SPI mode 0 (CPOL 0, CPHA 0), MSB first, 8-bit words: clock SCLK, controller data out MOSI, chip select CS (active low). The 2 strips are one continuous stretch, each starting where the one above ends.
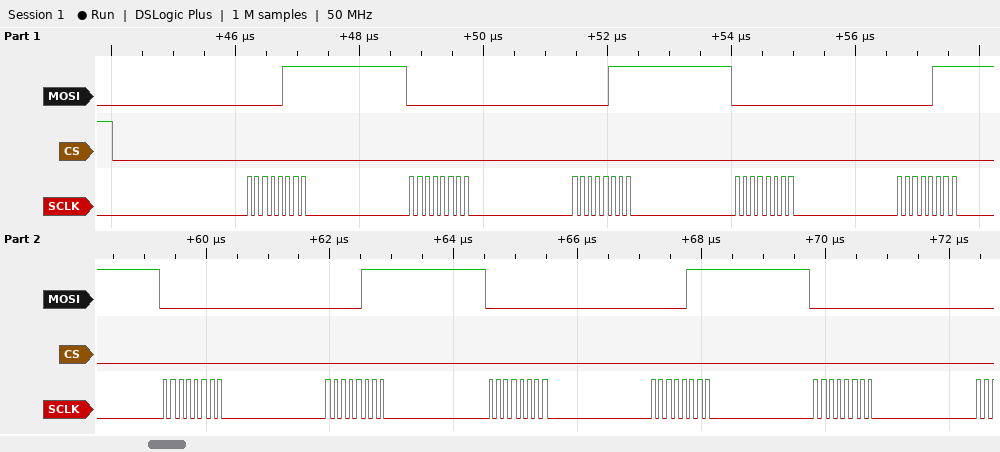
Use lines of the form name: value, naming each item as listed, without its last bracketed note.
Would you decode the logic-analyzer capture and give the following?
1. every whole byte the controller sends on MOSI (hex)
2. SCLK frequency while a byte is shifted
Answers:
every whole byte the controller sends on MOSI: 07 00 07 00 07 00 07 00 07 00
SCLK frequency while a byte is shifted: 8 MHz
